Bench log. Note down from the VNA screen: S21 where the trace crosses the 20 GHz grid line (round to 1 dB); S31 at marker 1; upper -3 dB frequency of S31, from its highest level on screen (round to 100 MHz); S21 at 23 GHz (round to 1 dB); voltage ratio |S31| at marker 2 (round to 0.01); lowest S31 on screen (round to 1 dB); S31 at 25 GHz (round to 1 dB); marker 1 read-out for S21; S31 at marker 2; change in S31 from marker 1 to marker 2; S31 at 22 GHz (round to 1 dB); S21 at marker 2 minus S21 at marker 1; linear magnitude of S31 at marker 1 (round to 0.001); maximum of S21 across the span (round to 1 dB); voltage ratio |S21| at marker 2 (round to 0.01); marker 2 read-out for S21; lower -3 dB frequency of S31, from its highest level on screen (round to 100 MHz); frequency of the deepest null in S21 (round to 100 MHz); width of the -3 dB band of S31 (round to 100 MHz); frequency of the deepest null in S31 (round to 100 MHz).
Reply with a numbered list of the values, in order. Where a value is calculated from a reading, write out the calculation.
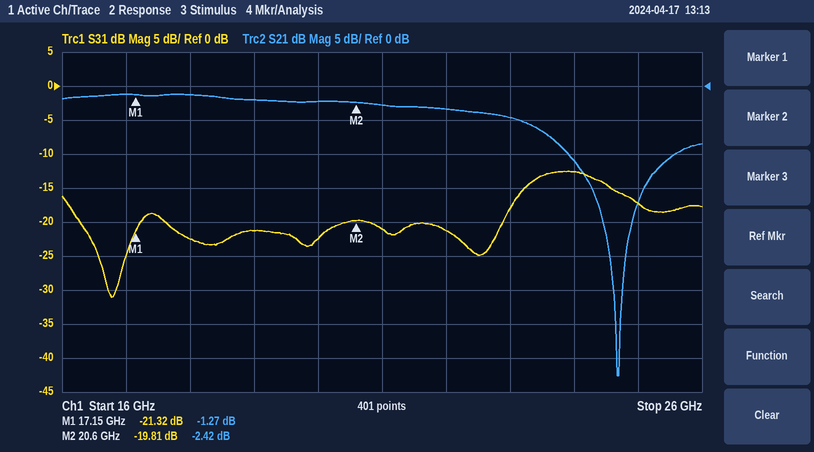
1. -2 dB
2. -21.32 dB
3. 24.7 GHz
4. -5 dB
5. 10^(-19.81/20) ≈ 0.10
6. -31 dB
7. -17 dB
8. -1.27 dB
9. -19.81 dB
10. -19.81 − (-21.32) = 1.51 dB
11. -21 dB
12. -2.42 − (-1.27) = -1.15 dB
13. 10^(-21.32/20) ≈ 0.086
14. -1 dB
15. 10^(-2.42/20) ≈ 0.76
16. -2.42 dB
17. 23.2 GHz
18. 24.7 GHz
19. 24.7 GHz − 23.2 GHz = 1.5 GHz
20. 16.8 GHz
